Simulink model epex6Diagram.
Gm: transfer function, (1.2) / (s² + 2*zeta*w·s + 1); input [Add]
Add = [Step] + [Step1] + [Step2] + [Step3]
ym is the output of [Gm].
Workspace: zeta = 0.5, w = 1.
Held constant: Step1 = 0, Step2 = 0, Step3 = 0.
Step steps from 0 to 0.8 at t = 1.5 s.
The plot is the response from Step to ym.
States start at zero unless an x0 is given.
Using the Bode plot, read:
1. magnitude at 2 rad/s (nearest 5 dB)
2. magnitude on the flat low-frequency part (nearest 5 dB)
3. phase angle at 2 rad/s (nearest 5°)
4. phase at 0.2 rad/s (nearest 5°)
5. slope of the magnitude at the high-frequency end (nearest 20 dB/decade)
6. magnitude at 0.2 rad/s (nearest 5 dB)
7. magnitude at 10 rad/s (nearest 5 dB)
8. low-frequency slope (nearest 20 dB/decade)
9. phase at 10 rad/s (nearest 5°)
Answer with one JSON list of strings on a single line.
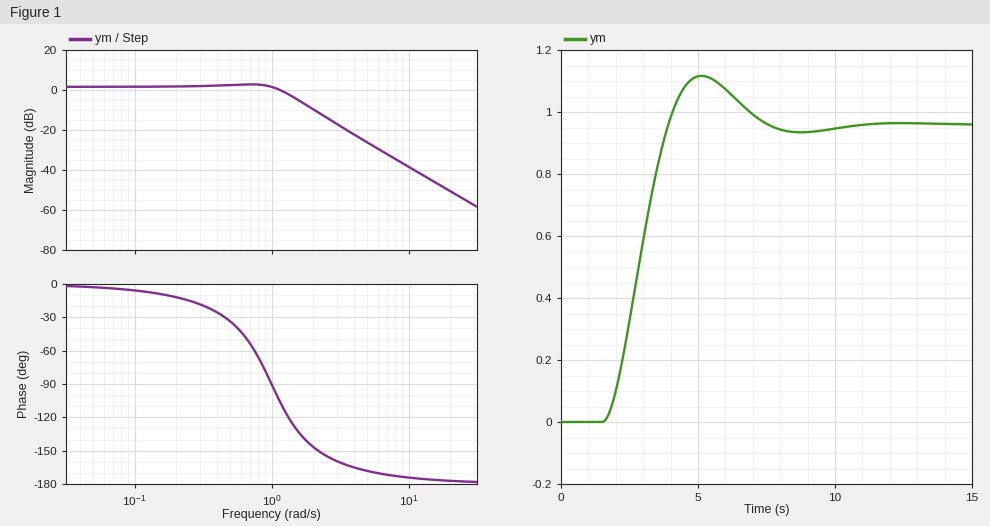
["-10 dB", "0 dB", "-145°", "-10°", "-40 dB/decade", "0 dB", "-40 dB", "0 dB/decade", "-175°"]
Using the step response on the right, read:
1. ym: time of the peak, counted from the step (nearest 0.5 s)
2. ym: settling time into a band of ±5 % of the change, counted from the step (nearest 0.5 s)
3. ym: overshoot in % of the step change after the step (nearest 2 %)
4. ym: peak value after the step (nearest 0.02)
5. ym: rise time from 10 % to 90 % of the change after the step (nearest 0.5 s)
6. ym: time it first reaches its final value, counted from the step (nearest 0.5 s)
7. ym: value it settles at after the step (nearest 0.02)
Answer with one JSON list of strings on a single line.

["3.5 s", "5.5 s", "16 %", "1.12", "1.5 s", "2.5 s", "0.96"]
